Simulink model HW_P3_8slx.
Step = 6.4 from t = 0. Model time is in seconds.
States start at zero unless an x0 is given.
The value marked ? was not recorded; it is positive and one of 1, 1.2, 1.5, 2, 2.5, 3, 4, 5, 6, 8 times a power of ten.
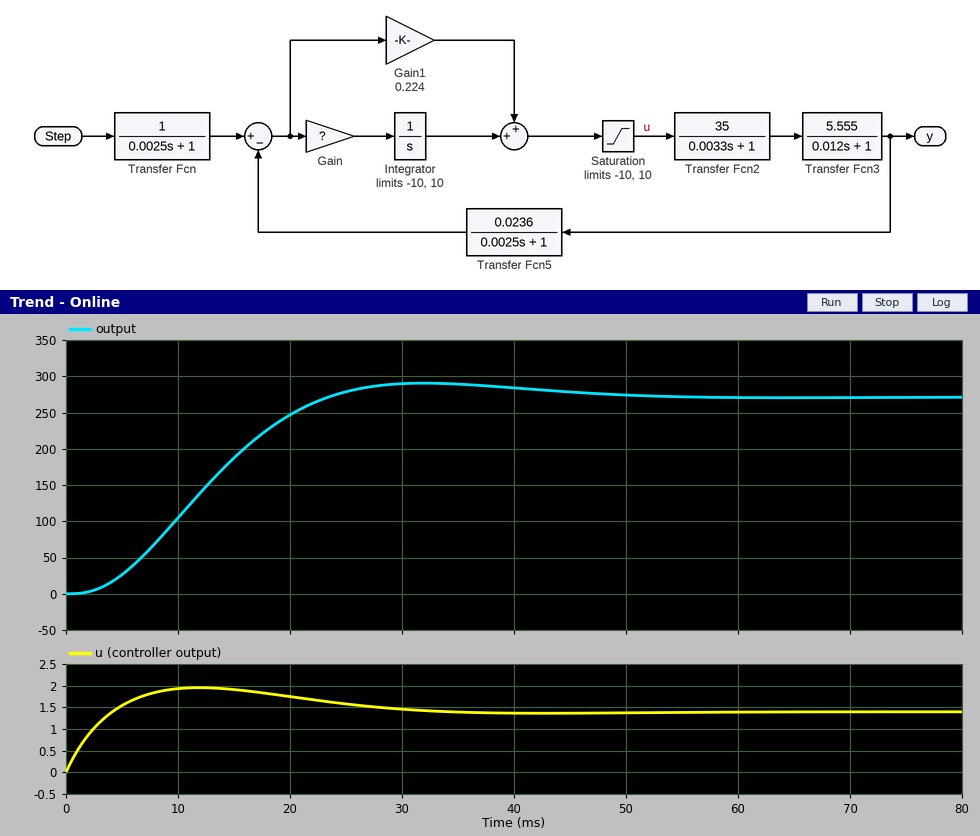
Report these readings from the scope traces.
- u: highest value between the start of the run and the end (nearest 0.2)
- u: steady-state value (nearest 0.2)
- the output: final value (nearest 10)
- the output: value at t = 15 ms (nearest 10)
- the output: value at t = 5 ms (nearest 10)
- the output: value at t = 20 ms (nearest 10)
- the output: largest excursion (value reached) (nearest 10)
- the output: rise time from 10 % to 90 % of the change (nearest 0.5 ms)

2.0
1.4
270
190
30
250
290
14.5 ms
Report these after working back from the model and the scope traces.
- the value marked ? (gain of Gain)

20
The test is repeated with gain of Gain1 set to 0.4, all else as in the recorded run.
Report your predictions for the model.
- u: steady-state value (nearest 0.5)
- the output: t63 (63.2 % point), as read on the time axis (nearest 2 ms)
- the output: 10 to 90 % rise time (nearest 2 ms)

1.5
10 ms
10 ms
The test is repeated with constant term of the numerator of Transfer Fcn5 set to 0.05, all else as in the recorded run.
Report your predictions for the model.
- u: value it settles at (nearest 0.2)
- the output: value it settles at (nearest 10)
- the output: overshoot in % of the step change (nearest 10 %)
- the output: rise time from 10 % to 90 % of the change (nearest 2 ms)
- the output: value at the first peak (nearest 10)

0.6
130
30 %
8 ms
170
